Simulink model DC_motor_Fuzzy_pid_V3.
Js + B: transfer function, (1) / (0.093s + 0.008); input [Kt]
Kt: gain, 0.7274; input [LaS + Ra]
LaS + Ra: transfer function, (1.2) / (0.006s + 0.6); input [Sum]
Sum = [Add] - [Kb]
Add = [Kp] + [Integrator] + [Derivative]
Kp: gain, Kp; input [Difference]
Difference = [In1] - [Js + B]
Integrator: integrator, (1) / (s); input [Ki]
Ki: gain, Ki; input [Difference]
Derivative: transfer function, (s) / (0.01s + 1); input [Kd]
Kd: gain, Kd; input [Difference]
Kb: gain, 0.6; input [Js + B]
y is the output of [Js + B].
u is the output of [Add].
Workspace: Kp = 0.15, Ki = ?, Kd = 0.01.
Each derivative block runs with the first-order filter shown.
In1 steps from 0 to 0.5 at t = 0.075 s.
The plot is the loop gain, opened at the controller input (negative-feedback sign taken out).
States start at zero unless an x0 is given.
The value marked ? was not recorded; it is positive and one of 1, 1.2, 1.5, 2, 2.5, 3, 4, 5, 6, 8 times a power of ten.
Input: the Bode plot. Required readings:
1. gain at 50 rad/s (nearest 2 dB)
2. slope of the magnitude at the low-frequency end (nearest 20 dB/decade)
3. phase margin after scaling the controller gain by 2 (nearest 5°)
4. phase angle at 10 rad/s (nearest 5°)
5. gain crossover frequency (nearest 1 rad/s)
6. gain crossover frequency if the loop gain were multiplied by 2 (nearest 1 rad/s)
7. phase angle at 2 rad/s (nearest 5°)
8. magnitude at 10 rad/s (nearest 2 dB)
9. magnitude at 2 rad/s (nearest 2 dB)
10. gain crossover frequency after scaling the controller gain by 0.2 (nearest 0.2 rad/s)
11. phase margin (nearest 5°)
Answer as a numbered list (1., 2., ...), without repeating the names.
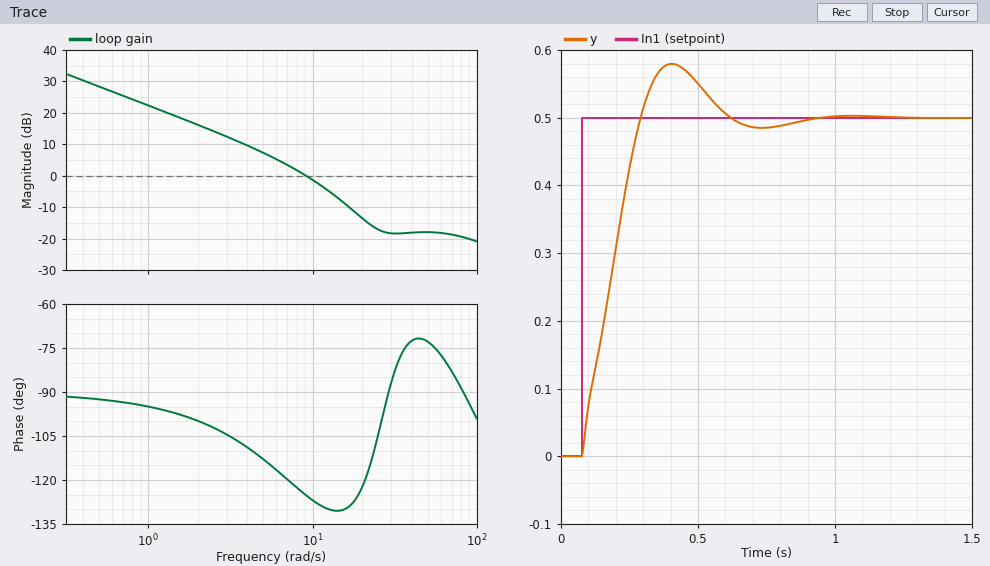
1. -18 dB
2. -20 dB/decade
3. 50°
4. -125°
5. 9 rad/s
6. 13 rad/s
7. -100°
8. -2 dB
9. 16 dB
10. 2.6 rad/s
11. 55°
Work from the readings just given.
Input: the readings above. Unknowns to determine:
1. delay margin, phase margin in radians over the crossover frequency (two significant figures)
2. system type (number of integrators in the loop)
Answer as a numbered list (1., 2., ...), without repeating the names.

1. 0.11 s
2. 1
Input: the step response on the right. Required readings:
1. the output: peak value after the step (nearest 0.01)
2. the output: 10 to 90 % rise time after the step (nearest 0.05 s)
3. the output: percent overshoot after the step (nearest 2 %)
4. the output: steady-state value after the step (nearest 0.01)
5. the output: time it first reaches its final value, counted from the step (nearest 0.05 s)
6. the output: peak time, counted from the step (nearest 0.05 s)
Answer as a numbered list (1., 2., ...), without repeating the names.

1. 0.58
2. 0.15 s
3. 16 %
4. 0.50
5. 0.20 s
6. 0.35 s
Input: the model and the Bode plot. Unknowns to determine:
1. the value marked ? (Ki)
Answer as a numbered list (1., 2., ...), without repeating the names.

1. 8
